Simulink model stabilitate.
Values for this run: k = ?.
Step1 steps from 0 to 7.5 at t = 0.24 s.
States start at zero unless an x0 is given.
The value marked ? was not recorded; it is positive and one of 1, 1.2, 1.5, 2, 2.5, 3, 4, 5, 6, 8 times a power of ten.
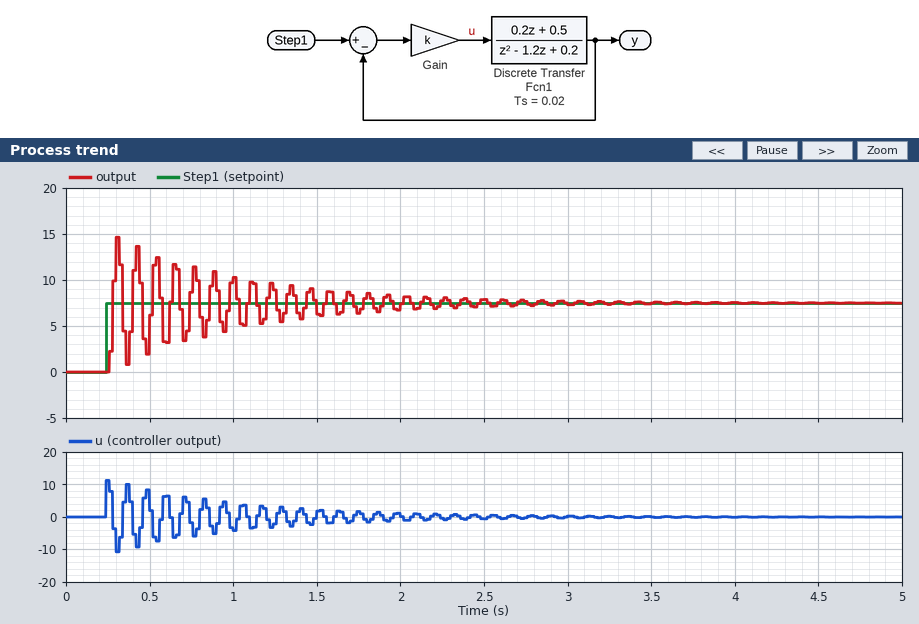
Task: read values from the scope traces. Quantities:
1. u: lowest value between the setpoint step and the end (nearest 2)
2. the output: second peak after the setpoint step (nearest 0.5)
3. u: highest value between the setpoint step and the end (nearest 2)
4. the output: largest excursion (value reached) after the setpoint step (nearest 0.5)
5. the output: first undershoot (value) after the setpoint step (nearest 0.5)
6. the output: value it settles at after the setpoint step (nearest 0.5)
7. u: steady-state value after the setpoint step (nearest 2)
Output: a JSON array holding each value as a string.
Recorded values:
["-10", "13.5", "12", "14.5", "1.0", "7.5", "0"]
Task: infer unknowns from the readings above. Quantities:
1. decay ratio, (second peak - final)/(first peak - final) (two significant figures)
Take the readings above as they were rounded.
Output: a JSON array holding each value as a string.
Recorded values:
["0.86"]
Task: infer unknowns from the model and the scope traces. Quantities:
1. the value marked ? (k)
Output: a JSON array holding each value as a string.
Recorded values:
["1.5"]
